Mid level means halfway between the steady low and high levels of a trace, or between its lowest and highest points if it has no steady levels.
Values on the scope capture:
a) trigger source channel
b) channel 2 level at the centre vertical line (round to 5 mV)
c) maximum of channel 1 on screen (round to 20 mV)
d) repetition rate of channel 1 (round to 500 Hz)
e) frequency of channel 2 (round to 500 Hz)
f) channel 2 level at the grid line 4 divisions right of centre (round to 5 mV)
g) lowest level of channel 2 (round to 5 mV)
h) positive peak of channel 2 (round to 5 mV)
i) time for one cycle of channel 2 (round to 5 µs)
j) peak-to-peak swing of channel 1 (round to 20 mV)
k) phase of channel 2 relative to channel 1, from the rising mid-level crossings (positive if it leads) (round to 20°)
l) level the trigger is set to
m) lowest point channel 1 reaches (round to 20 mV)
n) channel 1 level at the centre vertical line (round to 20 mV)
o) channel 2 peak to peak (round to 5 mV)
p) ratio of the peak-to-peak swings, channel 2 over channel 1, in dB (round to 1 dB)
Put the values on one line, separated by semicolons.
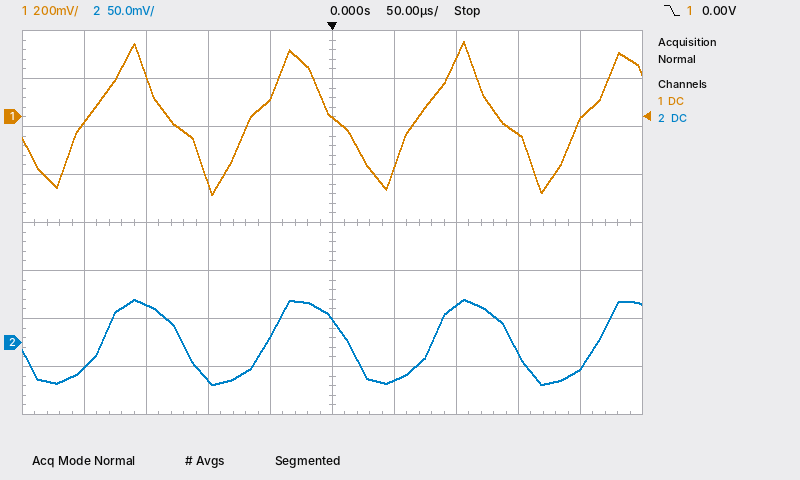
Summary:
channel 1; 25 mV; 320 mV; 7.5 kHz; 7.5 kHz; -25 mV; -45 mV; 45 mV; 135 µs; 640 mV; -40°; 0.00 V; -320 mV; 0 mV; 90 mV; -17 dB
